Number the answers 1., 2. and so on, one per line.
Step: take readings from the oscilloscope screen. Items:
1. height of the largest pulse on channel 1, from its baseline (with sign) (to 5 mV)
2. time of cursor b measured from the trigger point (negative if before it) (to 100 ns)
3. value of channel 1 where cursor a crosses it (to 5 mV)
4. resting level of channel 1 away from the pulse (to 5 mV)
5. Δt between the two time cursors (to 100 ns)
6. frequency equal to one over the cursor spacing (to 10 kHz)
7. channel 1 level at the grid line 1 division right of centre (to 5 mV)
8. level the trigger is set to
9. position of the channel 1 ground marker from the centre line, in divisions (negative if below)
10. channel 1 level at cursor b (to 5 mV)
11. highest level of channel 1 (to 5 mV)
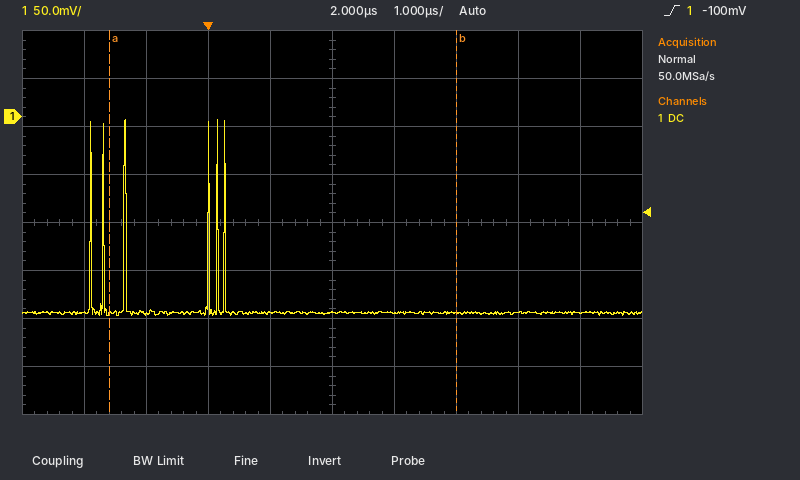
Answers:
1. +200 mV
2. +4.0 µs
3. -205 mV
4. -205 mV
5. 5.6 µs
6. 180 kHz
7. -205 mV
8. -100 mV
9. +2.2 div
10. -205 mV
11. -5 mV
